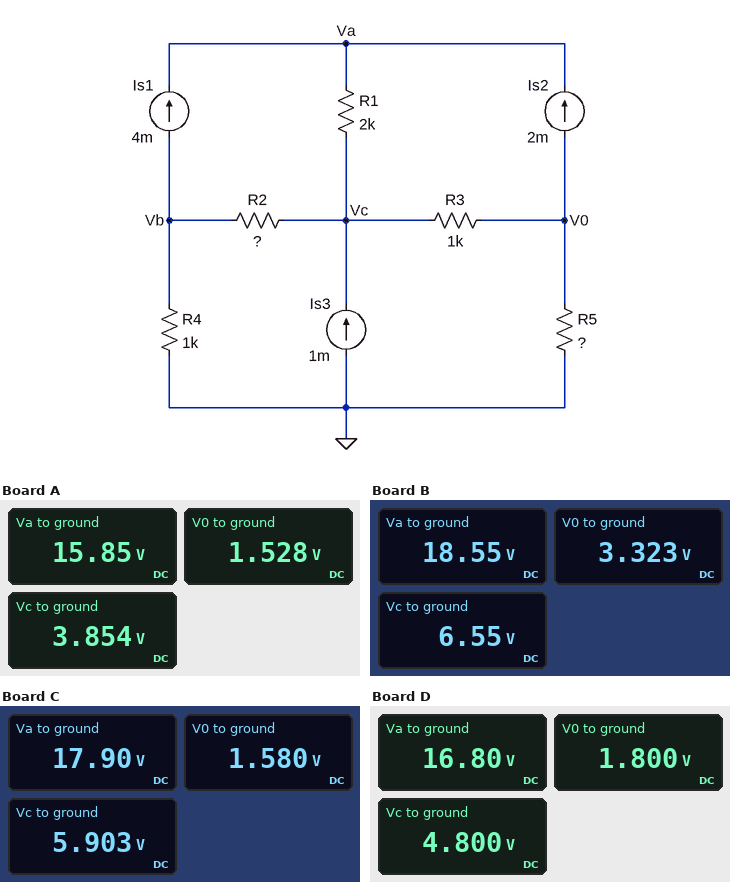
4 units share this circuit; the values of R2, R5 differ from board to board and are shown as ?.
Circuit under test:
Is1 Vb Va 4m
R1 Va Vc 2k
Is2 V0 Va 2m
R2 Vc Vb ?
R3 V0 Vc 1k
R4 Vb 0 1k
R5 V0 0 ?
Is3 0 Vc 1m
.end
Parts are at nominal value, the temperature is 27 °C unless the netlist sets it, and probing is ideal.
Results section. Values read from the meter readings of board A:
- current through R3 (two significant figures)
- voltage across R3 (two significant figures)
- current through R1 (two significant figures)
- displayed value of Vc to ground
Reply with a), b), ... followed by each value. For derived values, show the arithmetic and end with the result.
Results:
a) (3.854 V - 1.528 V) / 1 kΩ = 2.3 mA
b) 3.854 V - 1.528 V = 2.3 V
c) (15.85 V - 3.854 V) / 2 kΩ = 6.0 mA
d) 3.854 V
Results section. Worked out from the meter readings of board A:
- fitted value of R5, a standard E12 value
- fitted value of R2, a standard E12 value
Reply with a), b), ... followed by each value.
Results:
a) 4.7 kΩ
b) 680 Ω
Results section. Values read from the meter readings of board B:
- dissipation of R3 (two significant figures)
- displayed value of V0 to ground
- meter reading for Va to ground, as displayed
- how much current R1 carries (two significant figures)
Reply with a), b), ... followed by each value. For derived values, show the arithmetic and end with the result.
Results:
a) (6.55 V - 3.323 V)^2 / 1 kΩ = 10 mW
b) 3.323 V
c) 18.55 V
d) (18.55 V - 6.55 V) / 2 kΩ = 6.0 mA
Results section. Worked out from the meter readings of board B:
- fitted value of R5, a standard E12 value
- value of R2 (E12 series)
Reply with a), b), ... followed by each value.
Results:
a) 2.7 kΩ
b) 1.8 kΩ
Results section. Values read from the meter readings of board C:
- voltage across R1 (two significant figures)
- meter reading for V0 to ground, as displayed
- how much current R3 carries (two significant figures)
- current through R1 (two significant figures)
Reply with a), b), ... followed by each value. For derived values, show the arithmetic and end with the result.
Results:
a) 17.9 V - 5.903 V = 12 V
b) 1.580 V
c) (5.903 V - 1.58 V) / 1 kΩ = 4.3 mA
d) (17.9 V - 5.903 V) / 2 kΩ = 6.0 mA
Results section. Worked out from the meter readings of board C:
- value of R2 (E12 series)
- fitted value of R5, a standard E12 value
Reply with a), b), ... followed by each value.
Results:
a) 2.7 kΩ
b) 680 Ω
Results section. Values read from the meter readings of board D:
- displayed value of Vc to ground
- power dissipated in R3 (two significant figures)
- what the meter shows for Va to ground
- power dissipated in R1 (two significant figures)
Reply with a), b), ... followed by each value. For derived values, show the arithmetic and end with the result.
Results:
a) 4.800 V
b) (4.8 V - 1.8 V)^2 / 1 kΩ = 9.0 mW
c) 16.80 V
d) (16.8 V - 4.8 V)^2 / 2 kΩ = 72 mW
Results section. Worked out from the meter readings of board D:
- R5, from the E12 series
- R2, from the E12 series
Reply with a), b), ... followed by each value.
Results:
a) 1.8 kΩ
b) 1.2 kΩ
